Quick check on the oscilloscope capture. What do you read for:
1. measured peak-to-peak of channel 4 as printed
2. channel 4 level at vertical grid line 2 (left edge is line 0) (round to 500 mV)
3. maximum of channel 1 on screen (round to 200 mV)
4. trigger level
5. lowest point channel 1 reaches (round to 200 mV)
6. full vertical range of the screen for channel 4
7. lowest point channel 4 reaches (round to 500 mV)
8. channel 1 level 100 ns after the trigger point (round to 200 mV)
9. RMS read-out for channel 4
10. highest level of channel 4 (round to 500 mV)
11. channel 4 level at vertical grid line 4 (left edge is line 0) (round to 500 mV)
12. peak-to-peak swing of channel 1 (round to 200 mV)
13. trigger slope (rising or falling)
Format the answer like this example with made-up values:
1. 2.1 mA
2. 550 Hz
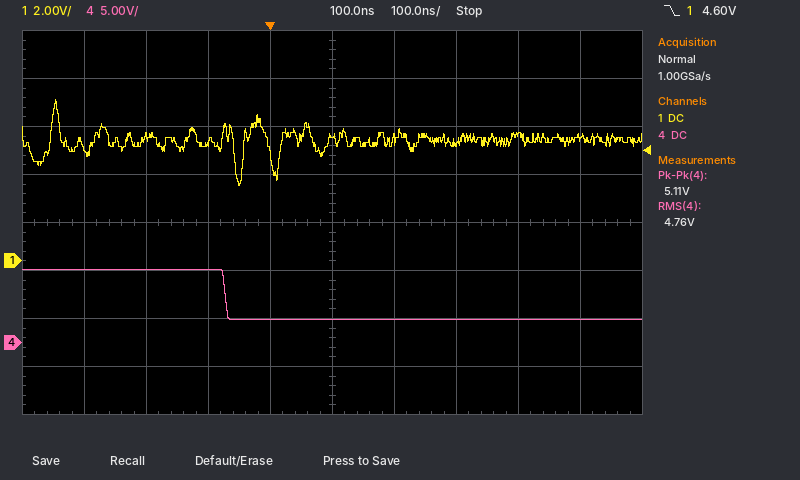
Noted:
1. 5.11 V
2. 7.5 V
3. 6.8 V
4. 4.60 V
5. 3.2 V
6. 40 V
7. 2.5 V
8. 5.2 V
9. 4.76 V
10. 7.5 V
11. 2.5 V
12. 3.6 V
13. falling
